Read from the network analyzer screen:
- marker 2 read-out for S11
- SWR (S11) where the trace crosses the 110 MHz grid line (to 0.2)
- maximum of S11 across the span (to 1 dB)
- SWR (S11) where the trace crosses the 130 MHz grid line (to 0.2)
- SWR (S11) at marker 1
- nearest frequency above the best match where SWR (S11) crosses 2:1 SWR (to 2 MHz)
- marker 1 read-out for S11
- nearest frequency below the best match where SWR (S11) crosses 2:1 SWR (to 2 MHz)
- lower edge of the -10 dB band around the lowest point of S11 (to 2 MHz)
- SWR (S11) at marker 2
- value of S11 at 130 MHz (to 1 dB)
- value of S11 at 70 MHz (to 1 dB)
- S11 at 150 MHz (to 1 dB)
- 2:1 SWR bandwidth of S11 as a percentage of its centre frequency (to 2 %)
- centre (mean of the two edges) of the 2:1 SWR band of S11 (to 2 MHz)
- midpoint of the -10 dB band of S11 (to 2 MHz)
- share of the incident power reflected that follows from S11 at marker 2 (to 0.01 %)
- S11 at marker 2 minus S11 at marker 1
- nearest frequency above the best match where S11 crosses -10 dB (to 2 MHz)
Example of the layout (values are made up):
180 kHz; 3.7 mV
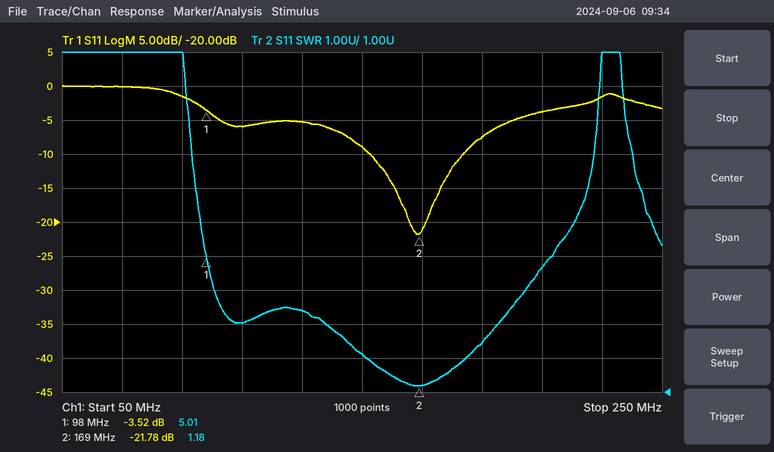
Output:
-21.78 dB; 3.0; 0 dB; 3.4; 5.01; 184 MHz; -3.52 dB; 152 MHz; 152 MHz; 1.18; -5 dB; 0 dB; -9 dB; 20 %; 168 MHz; 168 MHz; 0.66 %; -18.26 dB; 184 MHz
